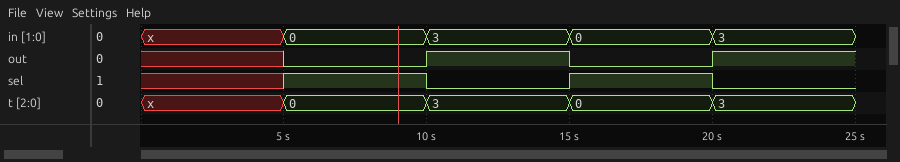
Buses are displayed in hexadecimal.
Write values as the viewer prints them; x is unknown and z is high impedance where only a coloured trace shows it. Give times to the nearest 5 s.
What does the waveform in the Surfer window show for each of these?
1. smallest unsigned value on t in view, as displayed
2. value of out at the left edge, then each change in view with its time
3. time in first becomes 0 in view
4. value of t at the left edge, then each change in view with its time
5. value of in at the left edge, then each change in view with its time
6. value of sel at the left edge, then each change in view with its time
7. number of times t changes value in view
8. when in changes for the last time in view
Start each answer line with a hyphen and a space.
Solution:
- 0
- x, 0 at 5 s, 1 at 10 s, 0 at 15 s, 1 at 20 s
- 5 s
- x, 0 at 5 s, 3 at 10 s, 0 at 15 s, 3 at 20 s
- x, 0 at 5 s, 3 at 10 s, 0 at 15 s, 3 at 20 s
- x, 1 at 5 s, 0 at 10 s, 1 at 15 s, 0 at 20 s
- 4
- 20 s
